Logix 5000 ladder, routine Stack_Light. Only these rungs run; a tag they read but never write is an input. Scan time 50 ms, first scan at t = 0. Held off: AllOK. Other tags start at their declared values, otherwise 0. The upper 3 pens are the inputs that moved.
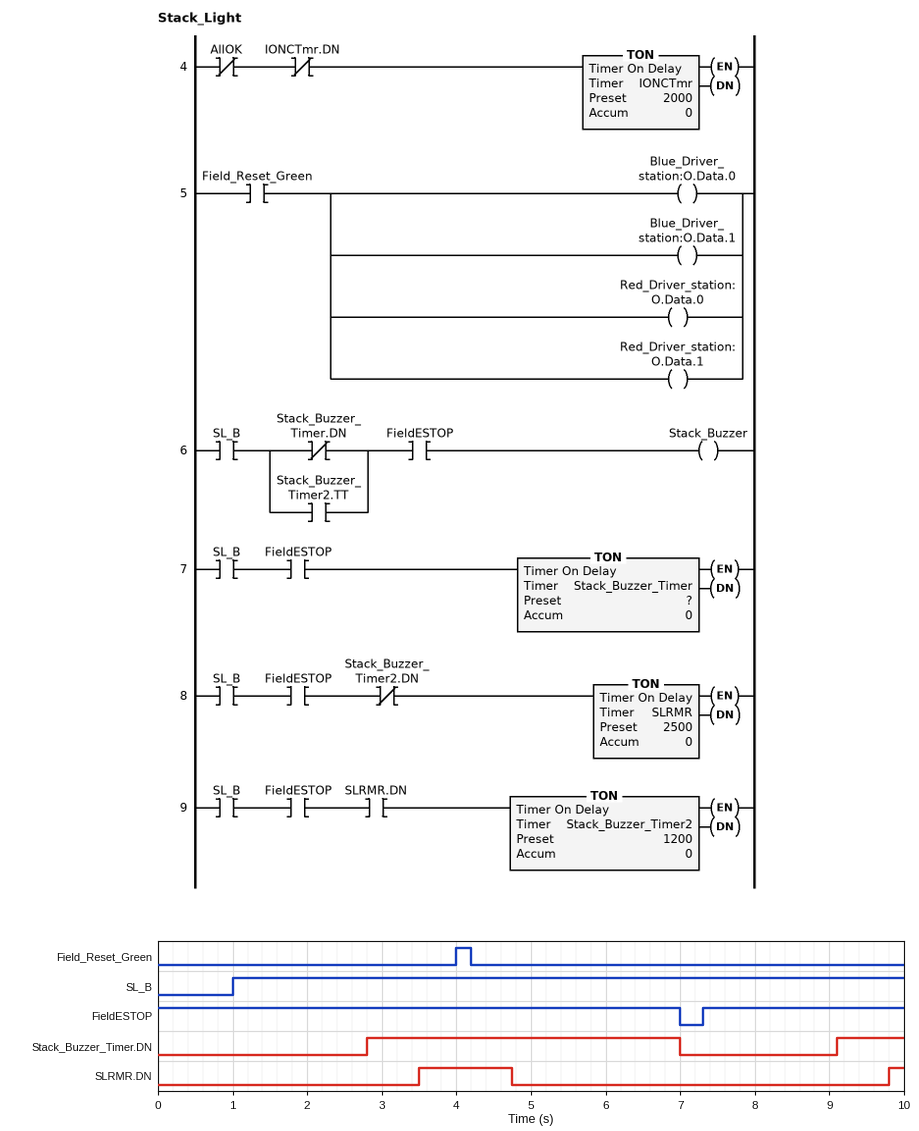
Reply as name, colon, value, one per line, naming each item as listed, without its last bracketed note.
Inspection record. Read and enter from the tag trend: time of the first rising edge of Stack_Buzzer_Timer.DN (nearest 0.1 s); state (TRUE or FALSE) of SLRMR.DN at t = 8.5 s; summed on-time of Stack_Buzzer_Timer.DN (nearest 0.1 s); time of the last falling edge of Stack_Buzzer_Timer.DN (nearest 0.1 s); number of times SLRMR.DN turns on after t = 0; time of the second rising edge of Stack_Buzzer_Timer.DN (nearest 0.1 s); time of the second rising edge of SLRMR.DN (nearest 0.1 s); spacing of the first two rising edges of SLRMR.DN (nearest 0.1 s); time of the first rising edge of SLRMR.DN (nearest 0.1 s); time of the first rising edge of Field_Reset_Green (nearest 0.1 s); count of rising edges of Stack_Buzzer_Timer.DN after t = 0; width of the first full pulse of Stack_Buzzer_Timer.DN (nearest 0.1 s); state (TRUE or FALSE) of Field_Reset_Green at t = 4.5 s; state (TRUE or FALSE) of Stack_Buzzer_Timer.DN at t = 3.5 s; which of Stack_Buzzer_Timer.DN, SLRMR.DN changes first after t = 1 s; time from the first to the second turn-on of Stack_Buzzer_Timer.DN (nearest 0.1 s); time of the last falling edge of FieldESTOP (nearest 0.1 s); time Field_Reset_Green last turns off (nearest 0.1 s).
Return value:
time of the first rising edge of Stack_Buzzer_Timer.DN: 2.8 s
state (TRUE or FALSE) of SLRMR.DN at t = 8.5 s: FALSE
summed on-time of Stack_Buzzer_Timer.DN: 5.1 s
time of the last falling edge of Stack_Buzzer_Timer.DN: 7.0 s
number of times SLRMR.DN turns on after t = 0: 2
time of the second rising edge of Stack_Buzzer_Timer.DN: 9.1 s
time of the second rising edge of SLRMR.DN: 9.8 s
spacing of the first two rising edges of SLRMR.DN: 6.3 s
time of the first rising edge of SLRMR.DN: 3.5 s
time of the first rising edge of Field_Reset_Green: 4.0 s
count of rising edges of Stack_Buzzer_Timer.DN after t = 0: 2
width of the first full pulse of Stack_Buzzer_Timer.DN: 4.2 s
state (TRUE or FALSE) of Field_Reset_Green at t = 4.5 s: FALSE
state (TRUE or FALSE) of Stack_Buzzer_Timer.DN at t = 3.5 s: TRUE
which of Stack_Buzzer_Timer.DN, SLRMR.DN changes first after t = 1 s: Stack_Buzzer_Timer.DN
time from the first to the second turn-on of Stack_Buzzer_Timer.DN: 6.3 s
time of the last falling edge of FieldESTOP: 7.0 s
time Field_Reset_Green last turns off: 4.2 s
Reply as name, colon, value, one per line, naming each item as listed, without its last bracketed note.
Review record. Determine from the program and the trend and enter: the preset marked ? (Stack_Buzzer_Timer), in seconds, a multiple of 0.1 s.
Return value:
the preset marked ? (Stack_Buzzer_Timer), in seconds, a multiple of 0.1 s: 1.8 s
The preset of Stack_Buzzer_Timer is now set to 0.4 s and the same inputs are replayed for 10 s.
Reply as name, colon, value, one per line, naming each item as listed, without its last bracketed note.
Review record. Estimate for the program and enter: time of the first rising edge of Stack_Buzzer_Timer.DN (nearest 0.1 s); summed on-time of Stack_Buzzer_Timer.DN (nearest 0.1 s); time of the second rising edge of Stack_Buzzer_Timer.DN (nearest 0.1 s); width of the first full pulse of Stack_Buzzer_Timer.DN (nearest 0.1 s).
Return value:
time of the first rising edge of Stack_Buzzer_Timer.DN: 1.4 s
summed on-time of Stack_Buzzer_Timer.DN: 7.9 s
time of the second rising edge of Stack_Buzzer_Timer.DN: 7.7 s
width of the first full pulse of Stack_Buzzer_Timer.DN: 5.6 s
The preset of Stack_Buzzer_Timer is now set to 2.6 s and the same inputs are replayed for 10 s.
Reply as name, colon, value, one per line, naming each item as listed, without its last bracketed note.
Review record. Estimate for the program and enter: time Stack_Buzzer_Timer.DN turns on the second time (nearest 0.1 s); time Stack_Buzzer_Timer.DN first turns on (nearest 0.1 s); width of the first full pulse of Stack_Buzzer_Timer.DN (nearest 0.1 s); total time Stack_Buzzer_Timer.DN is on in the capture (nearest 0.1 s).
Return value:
time Stack_Buzzer_Timer.DN turns on the second time: 9.9 s
time Stack_Buzzer_Timer.DN first turns on: 3.6 s
width of the first full pulse of Stack_Buzzer_Timer.DN: 3.4 s
total time Stack_Buzzer_Timer.DN is on in the capture: 3.5 s
